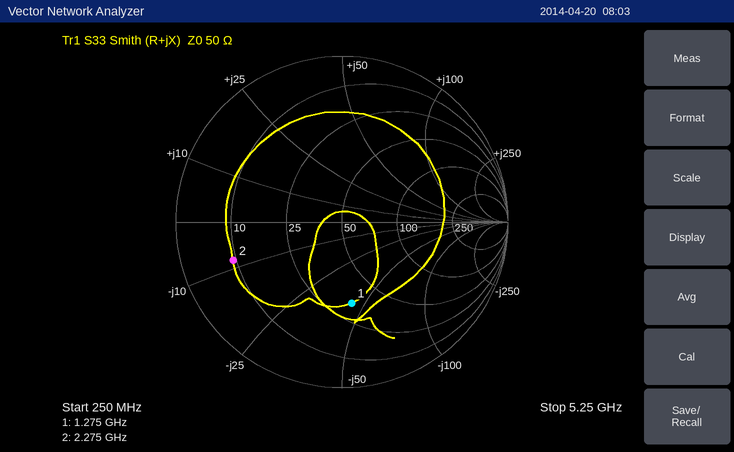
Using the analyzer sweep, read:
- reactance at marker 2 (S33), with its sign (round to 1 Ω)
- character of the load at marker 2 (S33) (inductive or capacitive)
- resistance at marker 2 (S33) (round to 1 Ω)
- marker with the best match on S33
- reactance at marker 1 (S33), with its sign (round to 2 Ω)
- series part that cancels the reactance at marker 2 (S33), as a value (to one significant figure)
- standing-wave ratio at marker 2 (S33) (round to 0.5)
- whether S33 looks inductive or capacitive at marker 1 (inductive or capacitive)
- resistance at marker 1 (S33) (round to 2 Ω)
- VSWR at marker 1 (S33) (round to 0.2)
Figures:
-8 Ω
capacitive
9 Ω
marker 1
-44 Ω
600 pH
5.5
capacitive
34 Ω
3.0
